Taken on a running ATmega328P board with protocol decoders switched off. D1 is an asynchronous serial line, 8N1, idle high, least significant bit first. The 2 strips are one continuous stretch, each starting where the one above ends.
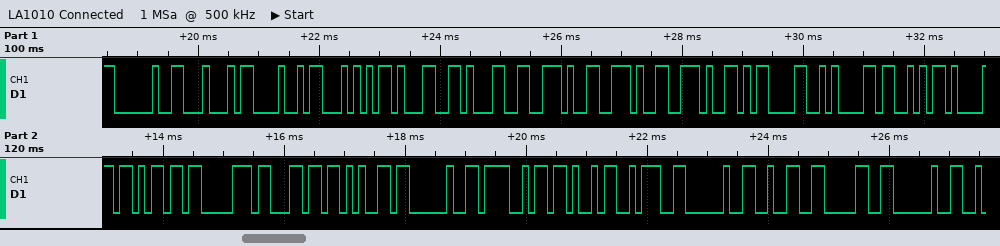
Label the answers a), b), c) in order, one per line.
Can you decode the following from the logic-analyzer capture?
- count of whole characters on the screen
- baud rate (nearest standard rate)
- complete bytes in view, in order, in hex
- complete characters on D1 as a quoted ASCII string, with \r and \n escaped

a) 25
b) 9600 baud
c) 20 44 48 54 31 31 2E 2E 2E 0D 0A 53 61 6D 70 6C 65 20 4F 4B 3A 20 32 30 20
d) " DHT11...\r\nSample OK: 20 "
